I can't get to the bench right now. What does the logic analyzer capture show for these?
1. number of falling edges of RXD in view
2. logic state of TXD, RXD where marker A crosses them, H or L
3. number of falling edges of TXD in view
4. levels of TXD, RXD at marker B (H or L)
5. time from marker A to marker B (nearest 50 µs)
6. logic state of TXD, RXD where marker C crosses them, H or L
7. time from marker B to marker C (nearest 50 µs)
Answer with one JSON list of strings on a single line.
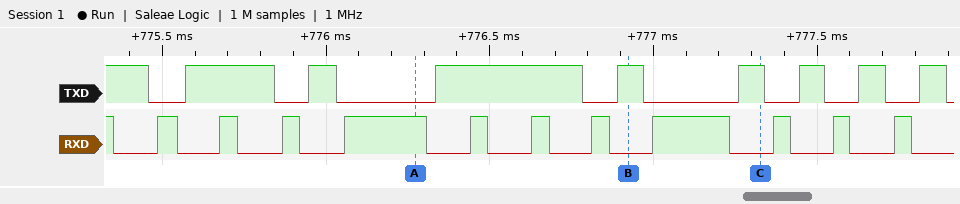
["12", "TXD=L, RXD=H", "9", "TXD=H, RXD=L", "650 µs", "TXD=H, RXD=L", "400 µs"]
